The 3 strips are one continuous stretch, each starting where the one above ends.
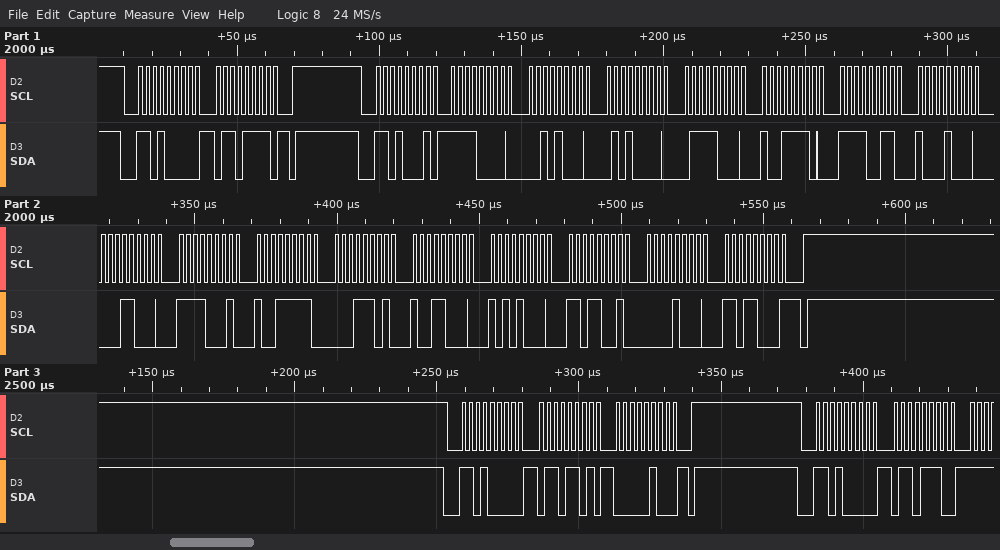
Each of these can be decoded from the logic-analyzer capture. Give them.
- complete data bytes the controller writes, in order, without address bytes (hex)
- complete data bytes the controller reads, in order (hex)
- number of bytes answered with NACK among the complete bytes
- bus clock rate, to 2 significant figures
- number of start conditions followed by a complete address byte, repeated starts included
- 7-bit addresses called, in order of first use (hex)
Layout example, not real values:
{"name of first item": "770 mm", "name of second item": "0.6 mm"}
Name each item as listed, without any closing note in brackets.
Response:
{"complete data bytes the controller writes, in order, without address bytes": "6F 6D 04 6E", "complete data bytes the controller reads, in order": "F0 28 50 78 9E F3 88 18 F1 9F 1D 98 A8 D9 08 D8", "number of bytes answered with NACK among the complete bytes": "1", "bus clock rate, to 2 significant figures": "400 kHz", "number of start conditions followed by a complete address byte, repeated starts included": "4", "7-bit addresses called, in order of first use": "0x68"}
